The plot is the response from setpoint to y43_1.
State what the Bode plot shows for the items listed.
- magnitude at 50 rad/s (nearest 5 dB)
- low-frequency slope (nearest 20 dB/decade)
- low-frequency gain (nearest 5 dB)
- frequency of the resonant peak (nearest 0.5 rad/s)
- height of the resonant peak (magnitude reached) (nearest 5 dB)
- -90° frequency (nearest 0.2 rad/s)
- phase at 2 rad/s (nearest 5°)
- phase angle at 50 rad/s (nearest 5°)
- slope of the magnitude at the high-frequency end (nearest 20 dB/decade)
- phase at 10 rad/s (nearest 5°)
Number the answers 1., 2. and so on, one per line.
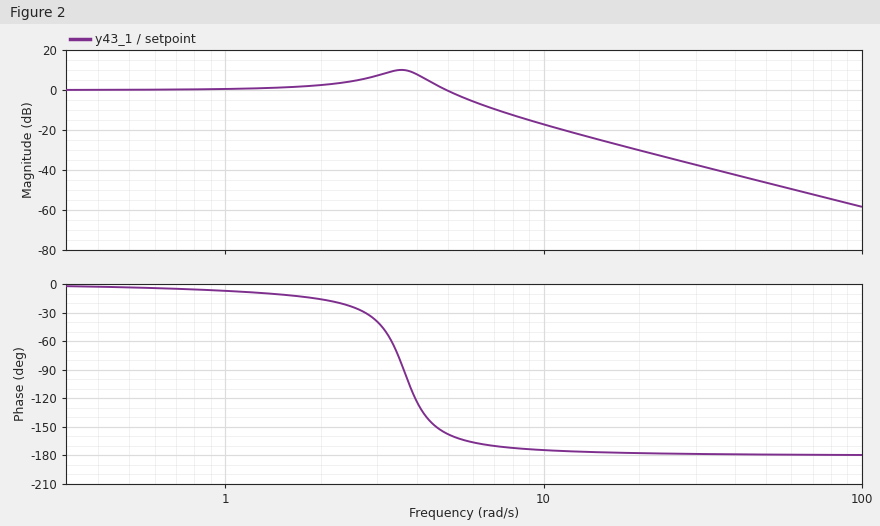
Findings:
1. -45 dB
2. 0 dB/decade
3. 0 dB
4. 3.5 rad/s
5. 10 dB
6. 3.6 rad/s
7. -15°
8. -180°
9. -40 dB/decade
10. -175°
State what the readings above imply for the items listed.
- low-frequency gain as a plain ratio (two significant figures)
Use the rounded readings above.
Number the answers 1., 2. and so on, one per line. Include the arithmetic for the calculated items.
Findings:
1. 10^(0 / 20) = 1.0
